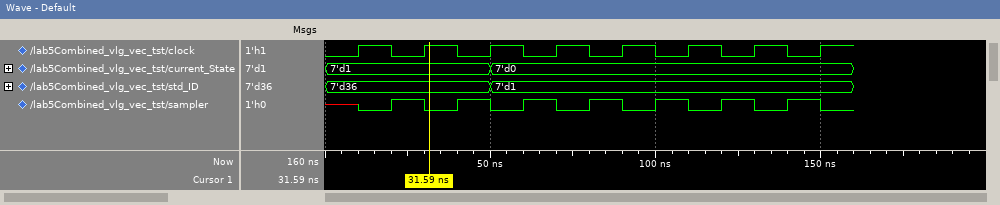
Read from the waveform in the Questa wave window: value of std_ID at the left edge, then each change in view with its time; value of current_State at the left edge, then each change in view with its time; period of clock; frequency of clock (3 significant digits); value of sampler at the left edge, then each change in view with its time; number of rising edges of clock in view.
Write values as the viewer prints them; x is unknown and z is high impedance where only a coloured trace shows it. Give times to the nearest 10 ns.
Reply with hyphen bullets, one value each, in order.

- 7'd36, 7'd1 at 50 ns
- 7'd1, 7'd0 at 50 ns
- 20 ns
- 50.0 MHz
- x, 0 at 10 ns, 1 at 20 ns, 0 at 30 ns, 1 at 40 ns, 0 at 50 ns, 1 at 60 ns, 0 at 70 ns, 1 at 80 ns, 0 at 90 ns, 1 at 100 ns, 0 at 110 ns, 1 at 120 ns, 0 at 130 ns, 1 at 140 ns, 0 at 150 ns
- 8
